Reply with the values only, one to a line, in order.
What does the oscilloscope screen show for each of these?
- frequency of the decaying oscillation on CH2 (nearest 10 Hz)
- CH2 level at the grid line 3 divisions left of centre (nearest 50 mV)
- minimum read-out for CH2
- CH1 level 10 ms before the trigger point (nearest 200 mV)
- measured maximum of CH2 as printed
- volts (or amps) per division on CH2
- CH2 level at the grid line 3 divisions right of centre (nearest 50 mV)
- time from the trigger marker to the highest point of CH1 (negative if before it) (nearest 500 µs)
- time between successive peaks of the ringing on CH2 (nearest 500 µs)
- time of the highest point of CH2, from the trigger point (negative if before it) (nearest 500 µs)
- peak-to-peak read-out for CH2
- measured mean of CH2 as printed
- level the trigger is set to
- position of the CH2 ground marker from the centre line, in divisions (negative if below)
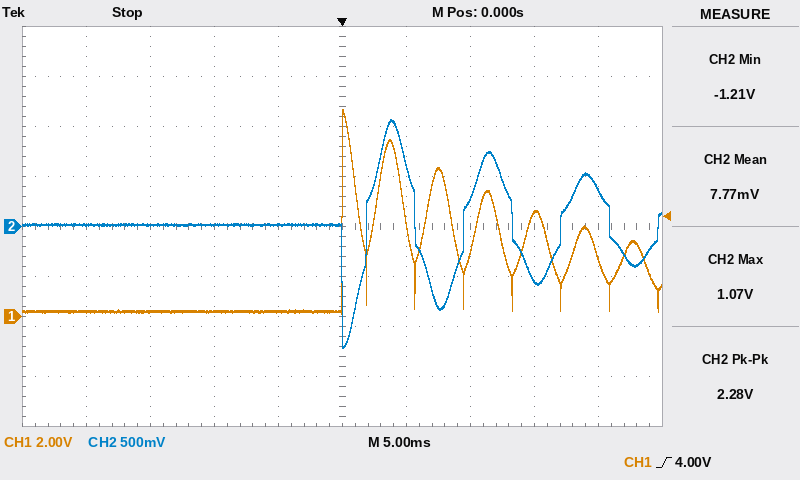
130 Hz
0 mV
-1.21 V
200 mV
1.07 V
500 mV
-550 mV
0.0 ms
7.5 ms
+4.0 ms
2.28 V
7.77 mV
4.00 V
0.0 div
